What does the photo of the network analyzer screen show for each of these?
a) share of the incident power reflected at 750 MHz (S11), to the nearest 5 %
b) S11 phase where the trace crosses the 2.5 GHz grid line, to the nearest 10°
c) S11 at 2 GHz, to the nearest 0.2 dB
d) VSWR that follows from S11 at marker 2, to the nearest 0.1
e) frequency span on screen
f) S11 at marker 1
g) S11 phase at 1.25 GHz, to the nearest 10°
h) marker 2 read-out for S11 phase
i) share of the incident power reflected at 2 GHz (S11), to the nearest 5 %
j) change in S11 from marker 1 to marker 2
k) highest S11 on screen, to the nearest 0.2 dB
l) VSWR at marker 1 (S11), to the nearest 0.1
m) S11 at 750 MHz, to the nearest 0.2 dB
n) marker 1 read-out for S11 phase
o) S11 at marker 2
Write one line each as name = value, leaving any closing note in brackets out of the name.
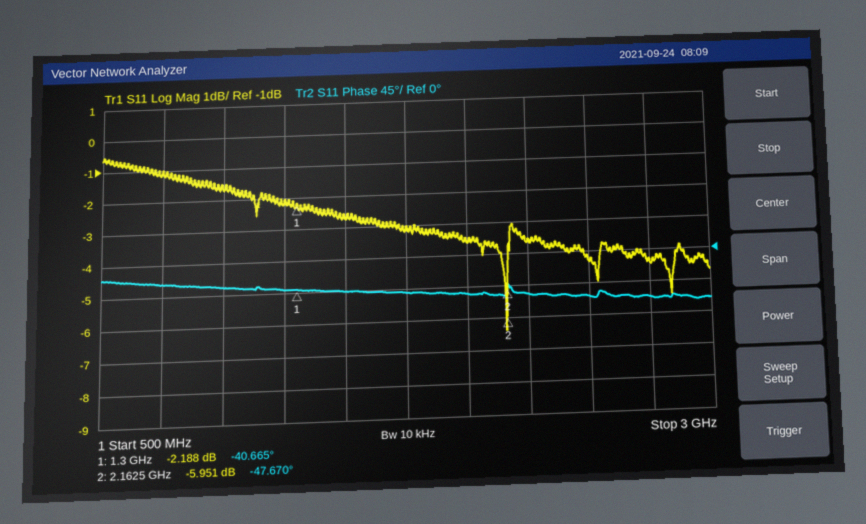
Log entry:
share of the incident power reflected at 750 MHz (S11), to the nearest 5 % = 80 %
S11 phase where the trace crosses the 2.5 GHz grid line, to the nearest 10° = -60°
S11 at 2 GHz, to the nearest 0.2 dB = -3.6 dB
VSWR that follows from S11 at marker 2, to the nearest 0.1 = 3.0
frequency span on screen = 2.5 GHz
S11 at marker 1 = -2.188 dB
S11 phase at 1.25 GHz, to the nearest 10° = -40°
marker 2 read-out for S11 phase = -47.670°
share of the incident power reflected at 2 GHz (S11), to the nearest 5 % = 45 %
change in S11 from marker 1 to marker 2 = -3.763 dB
highest S11 on screen, to the nearest 0.2 dB = -0.6 dB
VSWR at marker 1 (S11), to the nearest 0.1 = 8.0
S11 at 750 MHz, to the nearest 0.2 dB = -1.0 dB
marker 1 read-out for S11 phase = -40.665°
S11 at marker 2 = -5.951 dB
